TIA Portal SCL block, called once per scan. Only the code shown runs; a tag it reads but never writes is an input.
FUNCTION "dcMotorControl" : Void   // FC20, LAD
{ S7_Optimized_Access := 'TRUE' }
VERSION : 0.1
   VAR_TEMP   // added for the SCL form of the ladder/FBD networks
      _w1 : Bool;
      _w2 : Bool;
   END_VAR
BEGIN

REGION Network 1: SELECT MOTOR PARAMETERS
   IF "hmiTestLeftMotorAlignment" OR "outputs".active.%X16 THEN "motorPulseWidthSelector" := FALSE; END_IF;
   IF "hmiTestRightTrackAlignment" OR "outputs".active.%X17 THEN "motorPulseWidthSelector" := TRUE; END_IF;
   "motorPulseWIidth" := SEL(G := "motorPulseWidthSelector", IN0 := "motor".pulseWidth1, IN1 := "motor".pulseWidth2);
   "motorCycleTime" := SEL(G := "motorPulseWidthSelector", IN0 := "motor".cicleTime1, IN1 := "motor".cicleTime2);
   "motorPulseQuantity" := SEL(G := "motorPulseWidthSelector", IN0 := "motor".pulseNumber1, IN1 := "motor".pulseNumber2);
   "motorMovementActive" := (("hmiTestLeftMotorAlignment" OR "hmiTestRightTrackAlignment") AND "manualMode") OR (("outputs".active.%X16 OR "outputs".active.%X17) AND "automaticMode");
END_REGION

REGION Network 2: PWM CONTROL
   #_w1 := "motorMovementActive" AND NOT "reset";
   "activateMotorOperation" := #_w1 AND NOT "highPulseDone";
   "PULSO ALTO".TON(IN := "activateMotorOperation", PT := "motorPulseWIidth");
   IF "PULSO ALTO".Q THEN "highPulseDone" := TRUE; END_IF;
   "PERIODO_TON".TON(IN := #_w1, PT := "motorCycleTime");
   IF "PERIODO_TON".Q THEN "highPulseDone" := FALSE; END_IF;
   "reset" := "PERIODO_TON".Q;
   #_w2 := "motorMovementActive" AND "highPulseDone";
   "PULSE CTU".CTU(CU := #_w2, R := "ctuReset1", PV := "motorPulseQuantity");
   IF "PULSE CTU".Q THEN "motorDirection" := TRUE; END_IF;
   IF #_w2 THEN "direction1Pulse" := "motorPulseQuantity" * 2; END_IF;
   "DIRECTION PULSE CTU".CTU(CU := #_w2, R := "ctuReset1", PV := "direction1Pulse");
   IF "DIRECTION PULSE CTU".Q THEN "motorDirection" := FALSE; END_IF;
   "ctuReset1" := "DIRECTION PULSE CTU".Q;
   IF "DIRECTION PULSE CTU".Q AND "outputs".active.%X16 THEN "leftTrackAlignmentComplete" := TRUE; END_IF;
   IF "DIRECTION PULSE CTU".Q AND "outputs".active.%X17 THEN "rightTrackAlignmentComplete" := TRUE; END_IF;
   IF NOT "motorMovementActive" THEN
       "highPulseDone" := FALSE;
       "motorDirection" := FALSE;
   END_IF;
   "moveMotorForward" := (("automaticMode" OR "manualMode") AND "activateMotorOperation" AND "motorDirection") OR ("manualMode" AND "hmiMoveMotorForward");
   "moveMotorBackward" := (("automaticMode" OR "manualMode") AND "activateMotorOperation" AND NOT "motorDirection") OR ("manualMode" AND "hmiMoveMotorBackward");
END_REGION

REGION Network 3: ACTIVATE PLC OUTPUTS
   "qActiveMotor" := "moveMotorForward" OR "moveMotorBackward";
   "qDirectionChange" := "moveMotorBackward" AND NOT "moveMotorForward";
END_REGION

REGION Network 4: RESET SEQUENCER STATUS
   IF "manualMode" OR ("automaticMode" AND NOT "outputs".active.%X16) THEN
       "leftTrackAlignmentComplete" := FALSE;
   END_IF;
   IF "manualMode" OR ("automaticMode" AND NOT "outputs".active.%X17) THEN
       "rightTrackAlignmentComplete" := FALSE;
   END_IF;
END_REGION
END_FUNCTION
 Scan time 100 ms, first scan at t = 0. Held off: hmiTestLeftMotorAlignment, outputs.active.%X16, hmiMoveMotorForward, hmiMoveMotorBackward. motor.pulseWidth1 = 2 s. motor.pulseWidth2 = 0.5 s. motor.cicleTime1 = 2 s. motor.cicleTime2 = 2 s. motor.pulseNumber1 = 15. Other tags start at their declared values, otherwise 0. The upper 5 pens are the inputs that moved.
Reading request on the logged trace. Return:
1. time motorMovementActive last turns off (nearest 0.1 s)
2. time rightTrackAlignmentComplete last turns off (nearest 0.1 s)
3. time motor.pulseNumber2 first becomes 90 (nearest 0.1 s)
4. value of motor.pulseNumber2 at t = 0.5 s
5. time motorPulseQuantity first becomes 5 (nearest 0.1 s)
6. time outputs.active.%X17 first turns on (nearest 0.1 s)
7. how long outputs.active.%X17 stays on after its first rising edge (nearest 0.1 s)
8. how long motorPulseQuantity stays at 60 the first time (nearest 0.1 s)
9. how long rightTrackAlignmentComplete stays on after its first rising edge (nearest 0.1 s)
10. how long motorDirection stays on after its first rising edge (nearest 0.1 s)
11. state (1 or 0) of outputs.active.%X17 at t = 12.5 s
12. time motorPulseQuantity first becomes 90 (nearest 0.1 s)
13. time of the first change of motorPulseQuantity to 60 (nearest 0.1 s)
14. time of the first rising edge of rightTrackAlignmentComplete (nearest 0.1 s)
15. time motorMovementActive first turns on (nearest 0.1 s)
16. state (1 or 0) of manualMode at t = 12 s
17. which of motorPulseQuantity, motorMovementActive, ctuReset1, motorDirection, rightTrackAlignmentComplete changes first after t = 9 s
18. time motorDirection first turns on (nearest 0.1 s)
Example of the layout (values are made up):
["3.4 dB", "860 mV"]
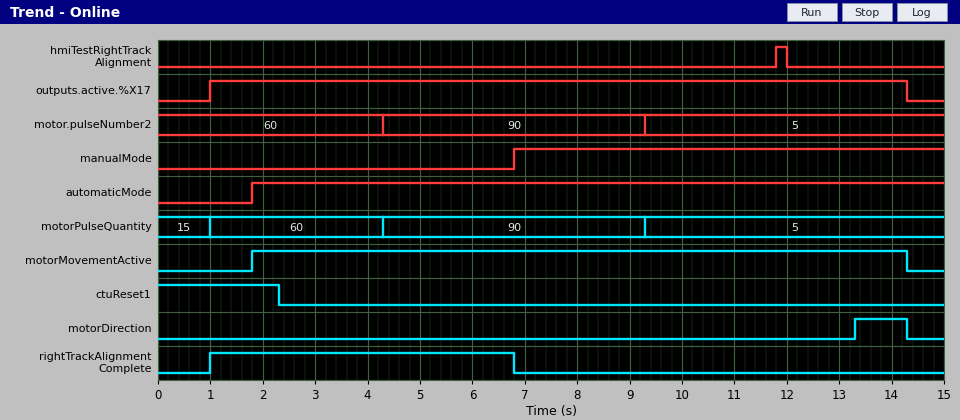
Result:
["14.3 s", "6.8 s", "4.3 s", "60", "9.3 s", "1.0 s", "13.3 s", "3.3 s", "5.8 s", "1.0 s", "1", "4.3 s", "1.0 s", "1.0 s", "1.8 s", "1", "motorPulseQuantity", "13.3 s"]
